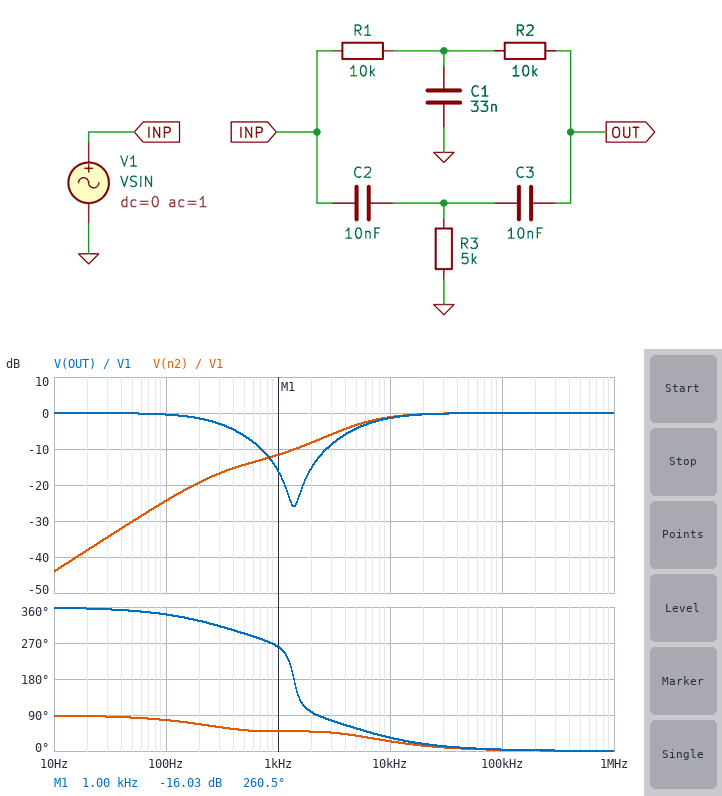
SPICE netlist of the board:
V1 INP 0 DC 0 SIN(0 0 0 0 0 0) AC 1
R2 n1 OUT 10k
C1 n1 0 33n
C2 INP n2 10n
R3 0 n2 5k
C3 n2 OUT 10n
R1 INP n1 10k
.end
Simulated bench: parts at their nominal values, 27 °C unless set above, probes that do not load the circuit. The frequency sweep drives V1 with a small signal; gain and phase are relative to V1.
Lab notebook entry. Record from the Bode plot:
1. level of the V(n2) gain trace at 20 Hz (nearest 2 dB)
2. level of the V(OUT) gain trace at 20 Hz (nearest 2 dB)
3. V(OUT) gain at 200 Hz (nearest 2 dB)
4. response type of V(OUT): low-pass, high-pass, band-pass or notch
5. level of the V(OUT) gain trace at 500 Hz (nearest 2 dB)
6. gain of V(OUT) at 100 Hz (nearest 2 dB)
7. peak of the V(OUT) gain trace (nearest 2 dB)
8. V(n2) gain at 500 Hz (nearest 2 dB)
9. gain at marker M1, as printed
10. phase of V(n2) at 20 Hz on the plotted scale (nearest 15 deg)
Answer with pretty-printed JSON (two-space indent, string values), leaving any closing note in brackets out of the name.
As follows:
{
  "level of the V(n2) gain trace at 20 Hz": "-38 dB",
  "level of the V(OUT) gain trace at 20 Hz": "0 dB",
  "V(OUT) gain at 200 Hz": "-2 dB",
  "response type of V(OUT): low-pass, high-pass, band-pass or notch": "notch",
  "level of the V(OUT) gain trace at 500 Hz": "-6 dB",
  "gain of V(OUT) at 100 Hz": "0 dB",
  "peak of the V(OUT) gain trace": "0 dB",
  "V(n2) gain at 500 Hz": "-14 dB",
  "gain at marker M1, as printed": "-16.03 dB",
  "phase of V(n2) at 20 Hz on the plotted scale": "90 deg"
}
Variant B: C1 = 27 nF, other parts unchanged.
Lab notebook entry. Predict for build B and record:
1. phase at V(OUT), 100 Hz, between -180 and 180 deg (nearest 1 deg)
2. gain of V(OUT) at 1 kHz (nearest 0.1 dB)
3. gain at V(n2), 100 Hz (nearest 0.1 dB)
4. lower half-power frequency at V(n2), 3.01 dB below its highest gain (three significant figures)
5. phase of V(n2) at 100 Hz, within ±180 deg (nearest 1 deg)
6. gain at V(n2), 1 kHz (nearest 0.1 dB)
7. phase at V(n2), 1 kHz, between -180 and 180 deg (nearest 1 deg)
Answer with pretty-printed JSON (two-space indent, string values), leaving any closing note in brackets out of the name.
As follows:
{
  "phase at V(OUT), 100 Hz, between -180 and 180 deg": "-17 deg",
  "gain of V(OUT) at 1 kHz": "-14.5 dB",
  "gain at V(n2), 100 Hz": "-24.3 dB",
  "lower half-power frequency at V(n2), 3.01 dB below its highest gain": "5.46 kHz",
  "phase of V(n2) at 100 Hz, within ±180 deg": "78 deg",
  "gain at V(n2), 1 kHz": "-11.3 dB",
  "phase at V(n2), 1 kHz, between -180 and 180 deg": "47 deg"
}
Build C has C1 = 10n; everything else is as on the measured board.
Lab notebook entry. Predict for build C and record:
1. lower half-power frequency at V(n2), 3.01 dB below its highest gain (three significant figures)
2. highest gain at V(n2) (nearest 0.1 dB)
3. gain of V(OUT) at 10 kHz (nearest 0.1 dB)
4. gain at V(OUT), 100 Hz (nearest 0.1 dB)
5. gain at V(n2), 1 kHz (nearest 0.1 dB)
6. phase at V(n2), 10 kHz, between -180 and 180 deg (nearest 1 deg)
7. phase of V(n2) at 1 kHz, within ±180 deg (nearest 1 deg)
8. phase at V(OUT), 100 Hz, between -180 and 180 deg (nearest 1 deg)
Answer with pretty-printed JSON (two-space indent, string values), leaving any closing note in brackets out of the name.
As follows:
{
  "lower half-power frequency at V(n2), 3.01 dB below its highest gain": "5.64 kHz",
  "highest gain at V(n2)": "0 dB",
  "gain of V(OUT) at 10 kHz": "-1.9 dB",
  "gain at V(OUT), 100 Hz": "-0.2 dB",
  "gain at V(n2), 1 kHz": "-9.8 dB",
  "phase at V(n2), 10 kHz, between -180 and 180 deg": "23 deg",
  "phase of V(n2) at 1 kHz, within ±180 deg": "45 deg",
  "phase at V(OUT), 100 Hz, between -180 and 180 deg": "-11 deg"
}
